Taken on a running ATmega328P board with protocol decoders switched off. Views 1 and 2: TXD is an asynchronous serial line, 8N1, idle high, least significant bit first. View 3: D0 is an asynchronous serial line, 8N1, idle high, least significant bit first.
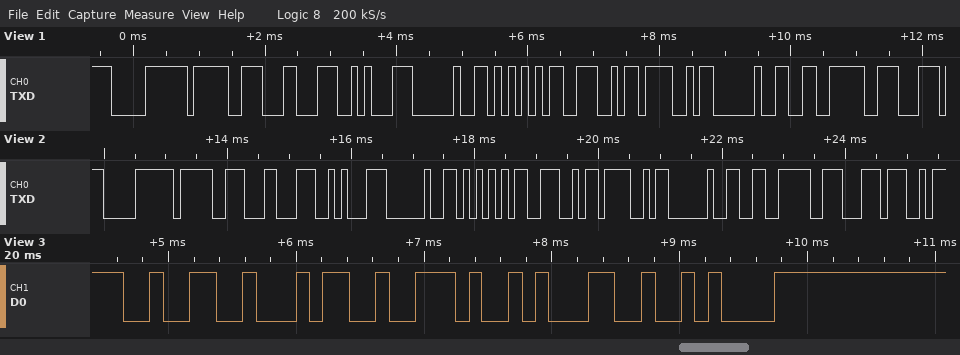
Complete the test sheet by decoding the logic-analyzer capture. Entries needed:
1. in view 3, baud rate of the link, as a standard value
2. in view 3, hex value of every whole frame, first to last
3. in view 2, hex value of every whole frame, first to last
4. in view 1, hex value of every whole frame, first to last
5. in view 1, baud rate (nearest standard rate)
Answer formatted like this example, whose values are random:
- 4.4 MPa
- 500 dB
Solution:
- 9600 baud
- 32 34 2E 31 0A
- F0 9F 8C 8A 20 55 4E 4F 20 E6 8E A7
- F0 9F 8C 8A 20 55 4E 4F 20 E6 8E
- 9600 baud
